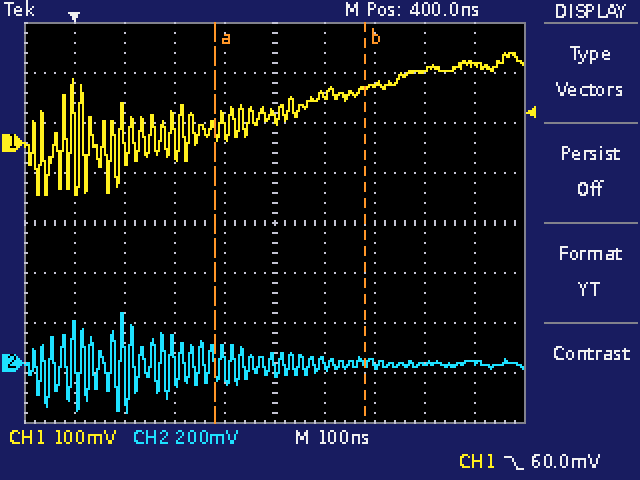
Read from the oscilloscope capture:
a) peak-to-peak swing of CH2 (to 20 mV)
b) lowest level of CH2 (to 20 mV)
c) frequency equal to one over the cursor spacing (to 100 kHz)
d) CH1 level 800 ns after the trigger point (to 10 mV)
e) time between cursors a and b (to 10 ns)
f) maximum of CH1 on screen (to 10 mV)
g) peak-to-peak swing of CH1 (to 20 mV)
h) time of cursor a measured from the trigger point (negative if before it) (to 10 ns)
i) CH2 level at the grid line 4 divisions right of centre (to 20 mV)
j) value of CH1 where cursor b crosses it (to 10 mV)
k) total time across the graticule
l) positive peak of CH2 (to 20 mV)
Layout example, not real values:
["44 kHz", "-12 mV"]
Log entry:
["400 mV", "-200 mV", "3.3 MHz", "160 mV", "300 ns", "180 mV", "280 mV", "+280 ns", "0 mV", "110 mV", "1 µs", "200 mV"]
